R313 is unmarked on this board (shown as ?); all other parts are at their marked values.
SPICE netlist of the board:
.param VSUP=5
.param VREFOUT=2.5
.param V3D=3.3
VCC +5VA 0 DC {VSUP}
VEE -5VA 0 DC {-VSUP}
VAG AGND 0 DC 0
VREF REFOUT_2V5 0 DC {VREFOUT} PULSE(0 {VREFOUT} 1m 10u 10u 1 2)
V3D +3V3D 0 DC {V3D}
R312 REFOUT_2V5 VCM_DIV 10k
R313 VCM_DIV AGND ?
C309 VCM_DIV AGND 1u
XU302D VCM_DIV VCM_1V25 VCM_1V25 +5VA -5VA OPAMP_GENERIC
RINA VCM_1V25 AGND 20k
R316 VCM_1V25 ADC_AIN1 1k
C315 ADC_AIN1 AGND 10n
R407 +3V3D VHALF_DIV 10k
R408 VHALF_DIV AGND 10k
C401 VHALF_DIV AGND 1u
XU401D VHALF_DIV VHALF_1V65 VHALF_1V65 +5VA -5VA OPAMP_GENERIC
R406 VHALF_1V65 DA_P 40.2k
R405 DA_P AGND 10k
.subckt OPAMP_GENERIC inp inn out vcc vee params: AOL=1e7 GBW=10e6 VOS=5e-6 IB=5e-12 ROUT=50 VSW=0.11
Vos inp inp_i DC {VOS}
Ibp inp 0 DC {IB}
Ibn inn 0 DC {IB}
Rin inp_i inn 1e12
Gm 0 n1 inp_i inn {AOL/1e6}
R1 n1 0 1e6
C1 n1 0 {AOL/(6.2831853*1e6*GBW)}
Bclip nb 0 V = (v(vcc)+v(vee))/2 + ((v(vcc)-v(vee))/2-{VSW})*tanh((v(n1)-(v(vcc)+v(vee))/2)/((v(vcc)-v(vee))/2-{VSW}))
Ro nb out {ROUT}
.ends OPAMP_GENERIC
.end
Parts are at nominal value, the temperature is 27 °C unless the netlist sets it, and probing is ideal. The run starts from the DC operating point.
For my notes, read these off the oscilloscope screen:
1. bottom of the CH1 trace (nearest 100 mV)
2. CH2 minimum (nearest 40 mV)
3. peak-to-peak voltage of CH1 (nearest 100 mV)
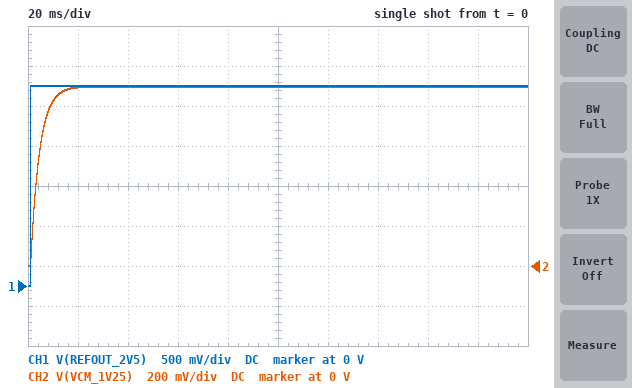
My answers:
0 V
0 V
2.5 V
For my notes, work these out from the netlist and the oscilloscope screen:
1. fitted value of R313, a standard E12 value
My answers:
5.6 kΩ
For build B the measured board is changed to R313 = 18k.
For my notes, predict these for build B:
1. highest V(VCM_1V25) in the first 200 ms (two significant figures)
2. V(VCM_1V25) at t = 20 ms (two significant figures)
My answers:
1.6 V
1.5 V
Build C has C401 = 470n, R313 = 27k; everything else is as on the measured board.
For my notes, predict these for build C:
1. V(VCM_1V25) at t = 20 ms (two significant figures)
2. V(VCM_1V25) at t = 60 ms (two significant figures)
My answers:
1.7 V
1.8 V
